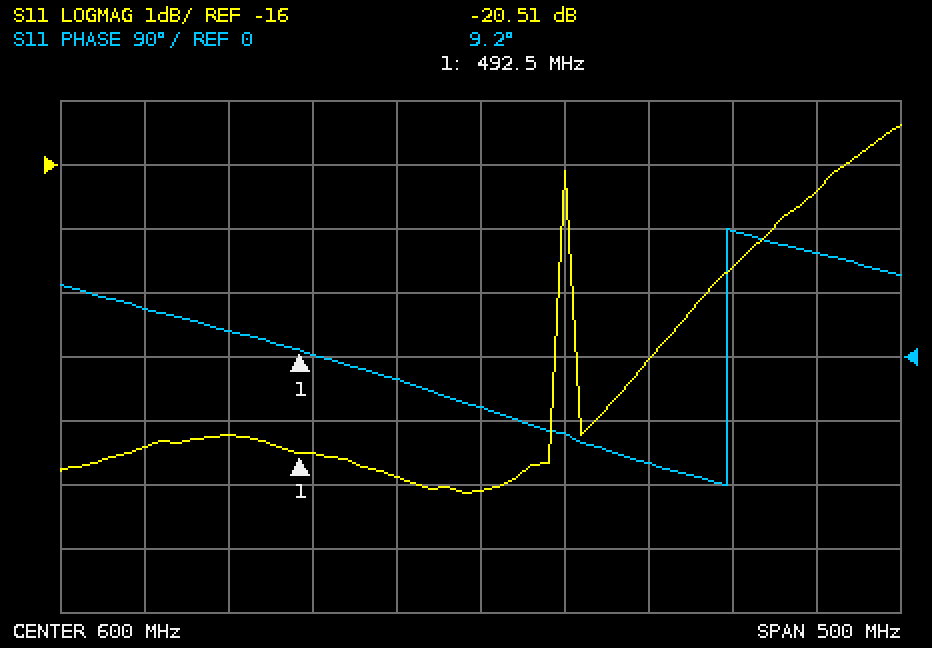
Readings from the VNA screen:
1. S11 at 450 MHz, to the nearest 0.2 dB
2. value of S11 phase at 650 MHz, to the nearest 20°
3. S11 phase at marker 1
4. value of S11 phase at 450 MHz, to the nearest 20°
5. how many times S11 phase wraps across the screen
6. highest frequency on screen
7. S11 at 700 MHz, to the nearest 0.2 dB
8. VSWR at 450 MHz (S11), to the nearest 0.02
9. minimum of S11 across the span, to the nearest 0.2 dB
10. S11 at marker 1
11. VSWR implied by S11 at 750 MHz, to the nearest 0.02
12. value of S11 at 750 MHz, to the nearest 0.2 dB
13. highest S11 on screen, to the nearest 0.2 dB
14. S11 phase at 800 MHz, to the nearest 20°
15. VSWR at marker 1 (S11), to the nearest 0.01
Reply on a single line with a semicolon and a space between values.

-20.2 dB; -100°; 9.2°; 40°; 1; 850 MHz; -19.0 dB; 1.22; -21.2 dB; -20.51 dB; 1.30; -17.6 dB; -15.4 dB; 140°; 1.21
